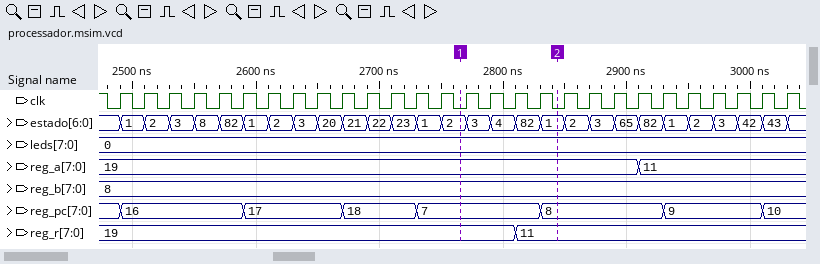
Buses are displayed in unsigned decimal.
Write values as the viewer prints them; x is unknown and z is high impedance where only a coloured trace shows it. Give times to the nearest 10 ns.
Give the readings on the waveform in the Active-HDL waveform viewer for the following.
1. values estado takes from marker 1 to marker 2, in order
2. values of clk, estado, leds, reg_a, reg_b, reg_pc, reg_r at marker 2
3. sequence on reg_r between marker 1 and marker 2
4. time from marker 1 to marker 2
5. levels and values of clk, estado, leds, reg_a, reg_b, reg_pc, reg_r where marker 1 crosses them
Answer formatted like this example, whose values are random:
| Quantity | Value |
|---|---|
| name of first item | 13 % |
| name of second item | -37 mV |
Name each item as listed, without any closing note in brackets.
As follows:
| Quantity | Value |
|---|---|
| values estado takes from marker 1 to marker 2, in order | 2, 3, 4, 82, 1 |
| values of clk, estado, leds, reg_a, reg_b, reg_pc, reg_r at marker 2 | clk=0, estado=1, leds=0, reg_a=19, reg_b=8, reg_pc=8, reg_r=11 |
| sequence on reg_r between marker 1 and marker 2 | 19, 11 |
| time from marker 1 to marker 2 | 80 ns |
| levels and values of clk, estado, leds, reg_a, reg_b, reg_pc, reg_r where marker 1 crosses them | clk=0, estado=2, leds=0, reg_a=19, reg_b=8, reg_pc=7, reg_r=19 |
